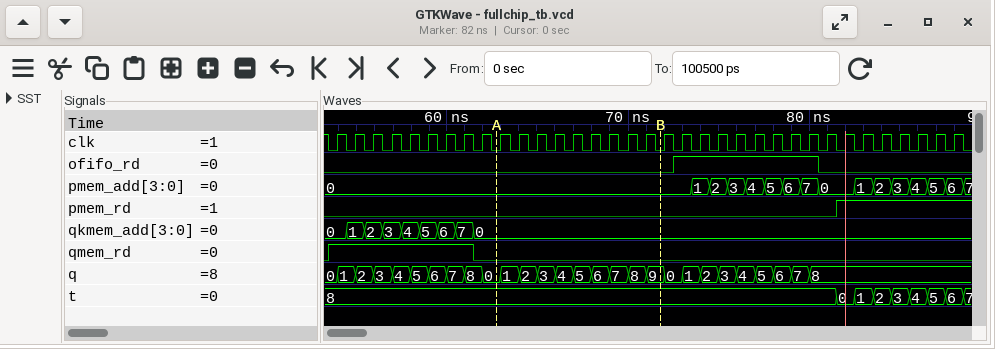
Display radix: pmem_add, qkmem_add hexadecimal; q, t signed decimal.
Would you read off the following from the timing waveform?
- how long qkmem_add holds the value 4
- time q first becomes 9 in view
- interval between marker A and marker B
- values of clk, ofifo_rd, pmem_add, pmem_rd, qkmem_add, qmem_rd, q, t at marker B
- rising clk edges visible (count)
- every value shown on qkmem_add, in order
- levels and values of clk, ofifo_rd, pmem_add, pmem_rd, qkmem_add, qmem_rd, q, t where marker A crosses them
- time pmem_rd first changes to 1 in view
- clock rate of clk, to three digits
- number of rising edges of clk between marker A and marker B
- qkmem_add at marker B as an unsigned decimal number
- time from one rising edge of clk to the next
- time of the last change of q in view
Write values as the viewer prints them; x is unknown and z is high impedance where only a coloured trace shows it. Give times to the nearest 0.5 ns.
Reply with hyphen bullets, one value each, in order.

- 1 ns
- 71 ns
- 9 ns
- clk=0, ofifo_rd=0, pmem_add=0, pmem_rd=0, qkmem_add=0, qmem_rd=0, q=9, t=8
- 35
- 0, 1, 2, 3, 4, 5, 6, 7, 0
- clk=0, ofifo_rd=0, pmem_add=0, pmem_rd=0, qkmem_add=0, qmem_rd=0, q=0, t=8
- 81.5 ns
- 1.00 GHz
- 9
- 0
- 1 ns
- 80 ns
